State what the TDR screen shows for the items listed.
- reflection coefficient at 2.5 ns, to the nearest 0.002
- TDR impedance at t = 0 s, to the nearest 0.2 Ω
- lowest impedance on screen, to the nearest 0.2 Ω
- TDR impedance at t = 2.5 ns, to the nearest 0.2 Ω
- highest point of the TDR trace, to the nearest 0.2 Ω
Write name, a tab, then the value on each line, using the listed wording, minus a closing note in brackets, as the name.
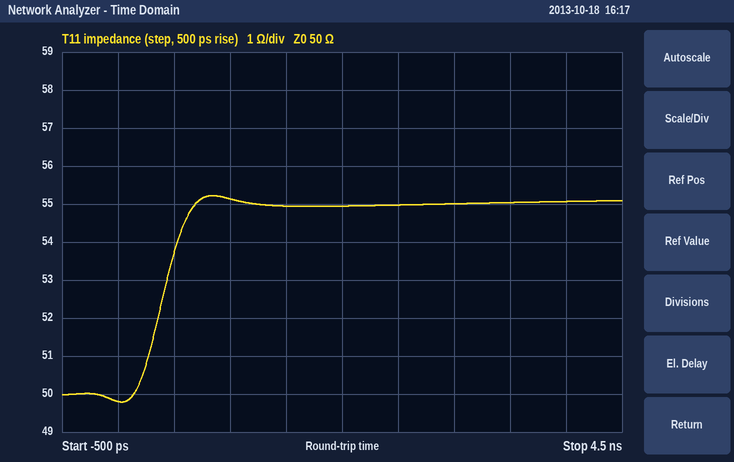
reflection coefficient at 2.5 ns, to the nearest 0.002	+0.048
TDR impedance at t = 0 s, to the nearest 0.2 Ω	49.8 Ω
lowest impedance on screen, to the nearest 0.2 Ω	49.8 Ω
TDR impedance at t = 2.5 ns, to the nearest 0.2 Ω	55.0 Ω
highest point of the TDR trace, to the nearest 0.2 Ω	55.2 Ω
